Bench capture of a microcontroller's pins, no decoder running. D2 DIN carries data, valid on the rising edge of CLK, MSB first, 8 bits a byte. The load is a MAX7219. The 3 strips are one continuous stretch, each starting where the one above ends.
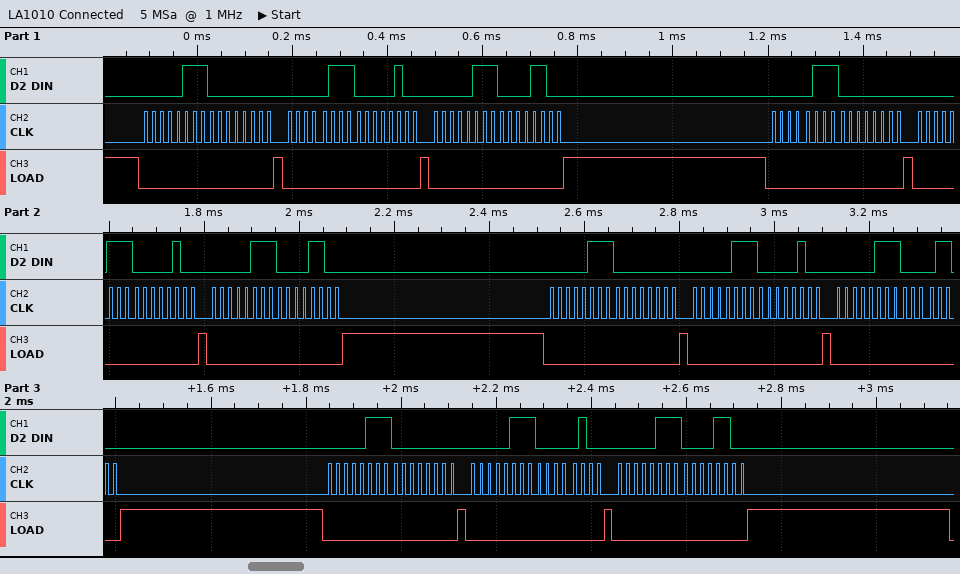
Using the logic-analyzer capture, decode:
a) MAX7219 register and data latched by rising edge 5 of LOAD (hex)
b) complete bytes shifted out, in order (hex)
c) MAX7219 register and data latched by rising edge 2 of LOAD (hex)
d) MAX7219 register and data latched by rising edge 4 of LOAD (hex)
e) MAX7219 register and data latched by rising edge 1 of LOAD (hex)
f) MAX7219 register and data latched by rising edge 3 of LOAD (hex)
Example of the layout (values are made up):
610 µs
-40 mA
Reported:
register 0x7, data 0x04
07 00 07 04 07 0C 07 00 07 04 07 0C 07 00 07 04 07 0C 07 00 07 04 07 0C
register 0x7, data 0x04
register 0x7, data 0x00
register 0x7, data 0x00
register 0x7, data 0x0C
